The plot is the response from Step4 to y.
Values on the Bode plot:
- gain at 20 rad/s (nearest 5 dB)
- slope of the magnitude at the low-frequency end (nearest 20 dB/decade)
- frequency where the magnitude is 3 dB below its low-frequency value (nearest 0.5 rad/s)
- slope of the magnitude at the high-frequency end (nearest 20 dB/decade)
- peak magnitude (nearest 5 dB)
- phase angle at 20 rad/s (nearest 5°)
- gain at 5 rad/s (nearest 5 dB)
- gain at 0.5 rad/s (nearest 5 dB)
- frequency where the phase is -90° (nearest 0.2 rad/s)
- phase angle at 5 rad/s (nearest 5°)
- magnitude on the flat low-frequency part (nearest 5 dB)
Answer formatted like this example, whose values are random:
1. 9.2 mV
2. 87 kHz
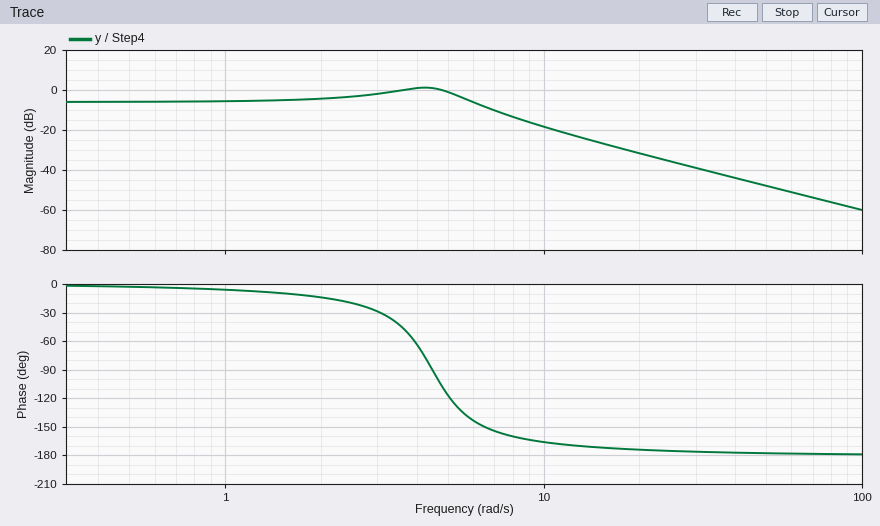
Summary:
1. -30 dB
2. 0 dB/decade
3. 6.5 rad/s
4. -40 dB/decade
5. 0 dB
6. -175°
7. 0 dB
8. -5 dB
9. 4.4 rad/s
10. -115°
11. -5 dB
